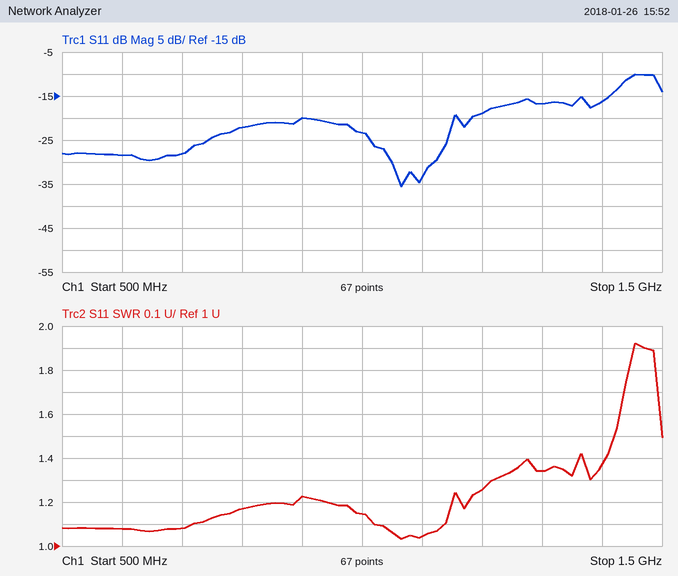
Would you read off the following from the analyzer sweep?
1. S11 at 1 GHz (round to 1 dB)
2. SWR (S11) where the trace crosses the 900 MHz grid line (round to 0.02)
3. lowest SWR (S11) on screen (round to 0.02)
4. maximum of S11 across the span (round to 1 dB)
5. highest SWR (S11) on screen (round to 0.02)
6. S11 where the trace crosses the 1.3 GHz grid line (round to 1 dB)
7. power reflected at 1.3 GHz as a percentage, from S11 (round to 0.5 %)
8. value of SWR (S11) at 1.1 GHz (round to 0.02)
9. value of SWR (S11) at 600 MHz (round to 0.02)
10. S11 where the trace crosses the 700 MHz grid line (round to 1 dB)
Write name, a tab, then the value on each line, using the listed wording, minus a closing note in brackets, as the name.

S11 at 1 GHz	-23 dB
SWR (S11) where the trace crosses the 900 MHz grid line	1.22
lowest SWR (S11) on screen	1.04
maximum of S11 across the span	-10 dB
highest SWR (S11) on screen	1.92
S11 where the trace crosses the 1.3 GHz grid line	-17 dB
power reflected at 1.3 GHz as a percentage, from S11	2.0 %
value of SWR (S11) at 1.1 GHz	1.04
value of SWR (S11) at 600 MHz	1.08
S11 where the trace crosses the 700 MHz grid line	-28 dB
